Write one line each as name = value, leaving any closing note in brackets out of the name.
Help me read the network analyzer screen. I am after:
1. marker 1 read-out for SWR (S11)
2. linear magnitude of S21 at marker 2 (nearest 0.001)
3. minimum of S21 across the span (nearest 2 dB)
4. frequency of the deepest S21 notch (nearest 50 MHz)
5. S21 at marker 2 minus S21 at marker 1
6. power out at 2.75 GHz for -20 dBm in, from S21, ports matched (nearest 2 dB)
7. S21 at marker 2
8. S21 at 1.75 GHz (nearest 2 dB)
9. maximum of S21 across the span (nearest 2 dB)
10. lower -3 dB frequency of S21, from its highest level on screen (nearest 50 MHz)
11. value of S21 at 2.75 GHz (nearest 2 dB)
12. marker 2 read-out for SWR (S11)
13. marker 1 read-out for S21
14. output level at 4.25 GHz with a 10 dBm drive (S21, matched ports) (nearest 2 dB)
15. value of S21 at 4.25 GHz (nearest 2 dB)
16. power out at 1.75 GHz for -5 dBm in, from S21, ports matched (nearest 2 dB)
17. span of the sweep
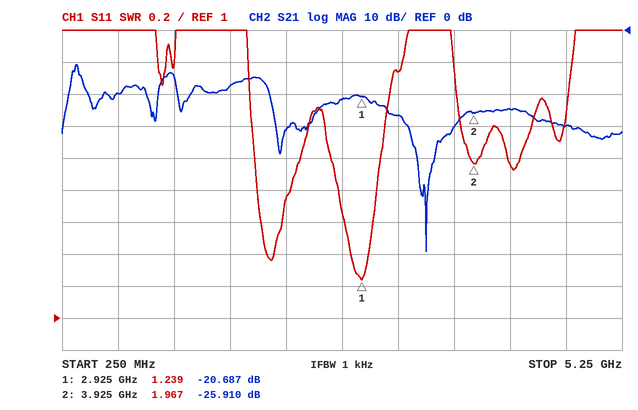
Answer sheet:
marker 1 read-out for SWR = 1.239
linear magnitude of S21 at marker 2 = 0.051
minimum of S21 across the span = -70 dB
frequency of the deepest S21 notch = 3.50 GHz
S21 at marker 2 minus S21 at marker 1 = -5.223 dB
power out at 2.75 GHz for -20 dBm in, from S21, ports matched = -42 dBm
S21 at marker 2 = -25.910 dB
S21 at 1.75 GHz = -18 dB
maximum of S21 across the span = -10 dB
lower -3 dB frequency of S21, from its highest level on screen = 350 MHz
value of S21 at 2.75 GHz = -22 dB
marker 2 read-out for SWR = 1.967
marker 1 read-out for S21 = -20.687 dB
output level at 4.25 GHz with a 10 dBm drive (S21, matched ports) = -14 dBm
value of S21 at 4.25 GHz = -24 dB
power out at 1.75 GHz for -5 dBm in, from S21, ports matched = -22 dBm
span of the sweep = 5 GHz
